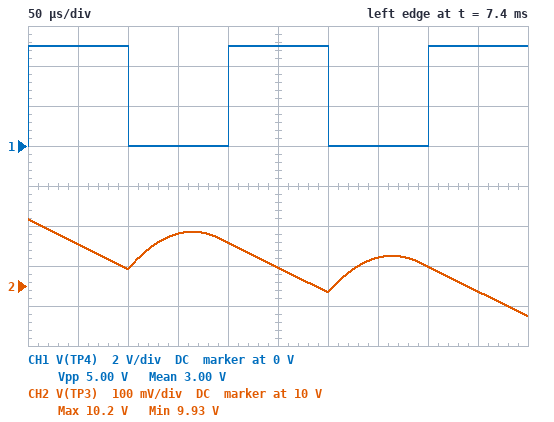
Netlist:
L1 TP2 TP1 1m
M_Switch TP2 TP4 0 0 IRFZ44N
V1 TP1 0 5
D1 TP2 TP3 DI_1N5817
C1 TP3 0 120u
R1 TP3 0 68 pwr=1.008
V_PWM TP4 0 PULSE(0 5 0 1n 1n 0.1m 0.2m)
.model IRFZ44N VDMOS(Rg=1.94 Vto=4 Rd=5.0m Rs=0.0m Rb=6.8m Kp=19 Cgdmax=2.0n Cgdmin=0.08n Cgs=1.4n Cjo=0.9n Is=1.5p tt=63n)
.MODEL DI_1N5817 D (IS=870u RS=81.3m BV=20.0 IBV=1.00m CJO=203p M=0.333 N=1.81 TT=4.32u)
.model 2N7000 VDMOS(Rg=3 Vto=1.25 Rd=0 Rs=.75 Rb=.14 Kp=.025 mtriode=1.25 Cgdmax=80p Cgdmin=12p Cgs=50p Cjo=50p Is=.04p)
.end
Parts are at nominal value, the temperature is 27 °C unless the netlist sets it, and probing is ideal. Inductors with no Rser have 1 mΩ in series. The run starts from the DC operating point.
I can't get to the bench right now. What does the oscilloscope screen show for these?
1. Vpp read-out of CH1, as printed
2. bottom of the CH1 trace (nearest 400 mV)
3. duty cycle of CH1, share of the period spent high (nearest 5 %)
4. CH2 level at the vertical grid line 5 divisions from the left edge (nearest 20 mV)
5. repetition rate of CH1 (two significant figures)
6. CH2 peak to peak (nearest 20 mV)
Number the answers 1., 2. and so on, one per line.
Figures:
1. 5.00 V
2. 0 V
3. 50 %
4. 10.04 V
5. 5.0 kHz
6. 240 mV
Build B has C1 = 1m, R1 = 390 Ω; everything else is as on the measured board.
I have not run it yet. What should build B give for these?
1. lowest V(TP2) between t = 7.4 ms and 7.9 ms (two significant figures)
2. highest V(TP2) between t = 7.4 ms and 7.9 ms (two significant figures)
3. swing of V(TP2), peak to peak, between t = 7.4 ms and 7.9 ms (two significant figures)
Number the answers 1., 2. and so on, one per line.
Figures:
1. -620 mV
2. 13 V
3. 14 V
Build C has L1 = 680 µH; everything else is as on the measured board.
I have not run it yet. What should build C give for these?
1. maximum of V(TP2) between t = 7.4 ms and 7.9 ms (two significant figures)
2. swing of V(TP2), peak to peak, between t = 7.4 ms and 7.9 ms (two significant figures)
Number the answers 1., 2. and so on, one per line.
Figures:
1. 11 V
2. 12 V
